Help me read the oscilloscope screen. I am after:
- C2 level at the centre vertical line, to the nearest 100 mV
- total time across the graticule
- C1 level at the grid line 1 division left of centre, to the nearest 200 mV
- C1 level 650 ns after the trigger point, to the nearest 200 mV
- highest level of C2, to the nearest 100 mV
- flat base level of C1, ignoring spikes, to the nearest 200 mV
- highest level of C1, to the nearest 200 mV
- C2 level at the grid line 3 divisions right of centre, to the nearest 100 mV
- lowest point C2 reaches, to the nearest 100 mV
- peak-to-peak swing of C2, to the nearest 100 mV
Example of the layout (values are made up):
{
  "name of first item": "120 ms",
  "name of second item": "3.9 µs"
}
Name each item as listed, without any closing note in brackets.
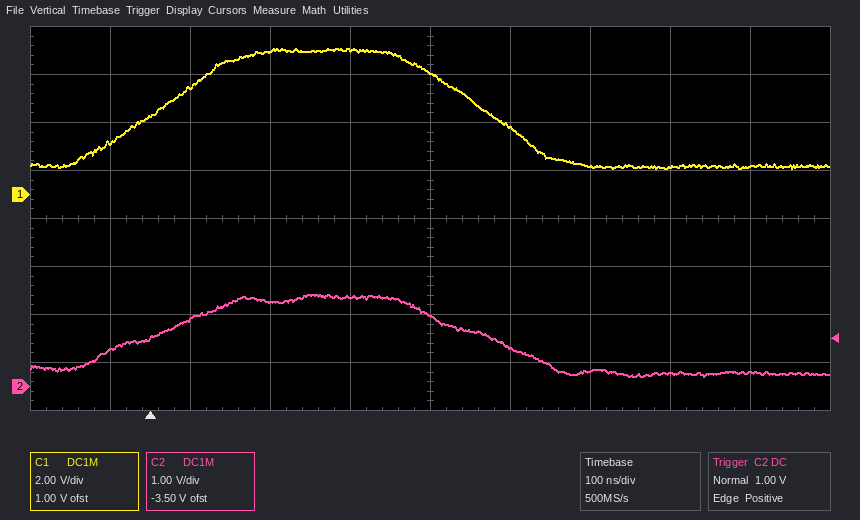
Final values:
{
  "C2 level at the centre vertical line, to the nearest 100 mV": "1.5 V",
  "total time across the graticule": "1 µs",
  "C1 level at the grid line 1 division left of centre, to the nearest 200 mV": "6.0 V",
  "C1 level 650 ns after the trigger point, to the nearest 200 mV": "1.2 V",
  "highest level of C2, to the nearest 100 mV": "1.9 V",
  "flat base level of C1, ignoring spikes, to the nearest 200 mV": "1.2 V",
  "highest level of C1, to the nearest 200 mV": "6.0 V",
  "C2 level at the grid line 3 divisions right of centre, to the nearest 100 mV": "300 mV",
  "lowest point C2 reaches, to the nearest 100 mV": "200 mV",
  "peak-to-peak swing of C2, to the nearest 100 mV": "1.7 V"
}
